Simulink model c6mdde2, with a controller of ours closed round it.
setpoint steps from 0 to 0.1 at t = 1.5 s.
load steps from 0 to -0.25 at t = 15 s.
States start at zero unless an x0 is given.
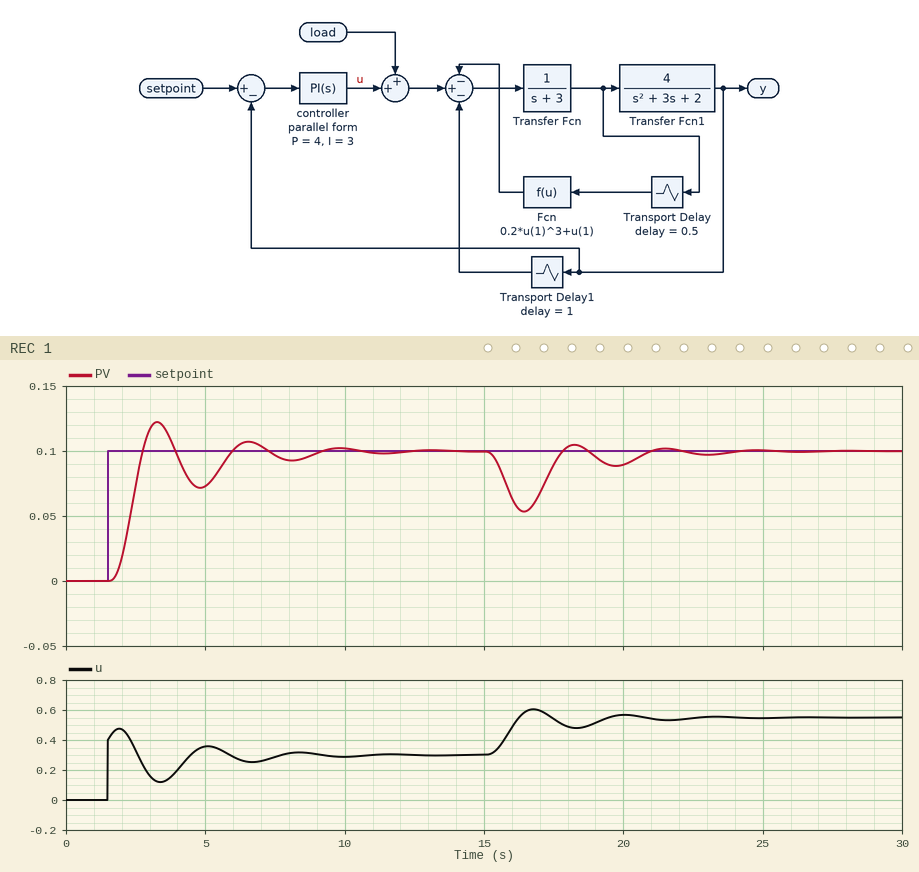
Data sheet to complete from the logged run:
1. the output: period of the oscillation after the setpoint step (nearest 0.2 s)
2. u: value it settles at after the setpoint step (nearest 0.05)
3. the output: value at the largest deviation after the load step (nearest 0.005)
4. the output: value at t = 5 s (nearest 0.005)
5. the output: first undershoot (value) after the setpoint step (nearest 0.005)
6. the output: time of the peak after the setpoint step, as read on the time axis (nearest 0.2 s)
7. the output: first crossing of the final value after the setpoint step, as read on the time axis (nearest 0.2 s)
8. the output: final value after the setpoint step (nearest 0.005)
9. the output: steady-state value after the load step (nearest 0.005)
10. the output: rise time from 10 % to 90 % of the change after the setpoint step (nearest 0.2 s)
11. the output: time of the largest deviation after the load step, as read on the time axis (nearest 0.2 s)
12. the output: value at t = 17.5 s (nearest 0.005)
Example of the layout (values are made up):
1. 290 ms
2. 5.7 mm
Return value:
1. 3.2 s
2. 0.30
3. 0.055
4. 0.075
5. 0.070
6. 3.2 s
7. 2.8 s
8. 0.100
9. 0.100
10. 0.8 s
11. 16.4 s
12. 0.090
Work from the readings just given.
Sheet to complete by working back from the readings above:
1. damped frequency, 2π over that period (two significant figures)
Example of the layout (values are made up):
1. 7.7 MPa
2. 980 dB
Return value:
1. 2.0 rad/s
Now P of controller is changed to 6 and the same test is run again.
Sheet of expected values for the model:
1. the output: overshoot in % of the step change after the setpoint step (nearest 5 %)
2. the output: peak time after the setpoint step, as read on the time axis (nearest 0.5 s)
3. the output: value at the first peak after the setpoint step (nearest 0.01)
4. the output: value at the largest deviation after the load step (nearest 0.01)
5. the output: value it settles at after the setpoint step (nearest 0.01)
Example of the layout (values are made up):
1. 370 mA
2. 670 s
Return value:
1. 30 %
2. 3.0 s
3. 0.13
4. 0.06
5. 0.10
